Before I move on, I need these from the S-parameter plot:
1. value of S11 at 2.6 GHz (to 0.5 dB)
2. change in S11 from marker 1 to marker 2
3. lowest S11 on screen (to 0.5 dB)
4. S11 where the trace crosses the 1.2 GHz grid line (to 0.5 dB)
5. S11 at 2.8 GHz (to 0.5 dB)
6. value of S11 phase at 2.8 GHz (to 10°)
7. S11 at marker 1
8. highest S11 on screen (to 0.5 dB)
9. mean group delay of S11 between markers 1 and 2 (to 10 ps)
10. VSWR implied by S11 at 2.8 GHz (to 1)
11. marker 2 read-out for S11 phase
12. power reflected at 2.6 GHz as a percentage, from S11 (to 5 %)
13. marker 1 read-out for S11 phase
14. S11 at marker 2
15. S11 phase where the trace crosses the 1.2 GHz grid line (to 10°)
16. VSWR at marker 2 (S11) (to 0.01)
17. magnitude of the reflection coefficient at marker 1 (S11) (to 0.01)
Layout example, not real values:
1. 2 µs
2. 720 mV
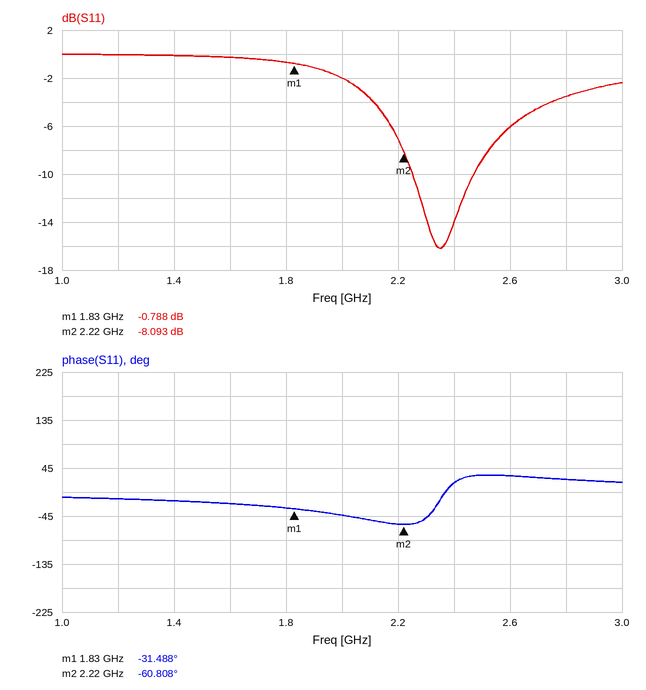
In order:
1. -6.0 dB
2. -7.305 dB
3. -16.0 dB
4. 0.0 dB
5. -3.5 dB
6. 20°
7. -0.788 dB
8. 0.0 dB
9. 210 ps
10. 5
11. -60.808°
12. 25 %
13. -31.488°
14. -8.093 dB
15. -10°
16. 2.30
17. 0.91
